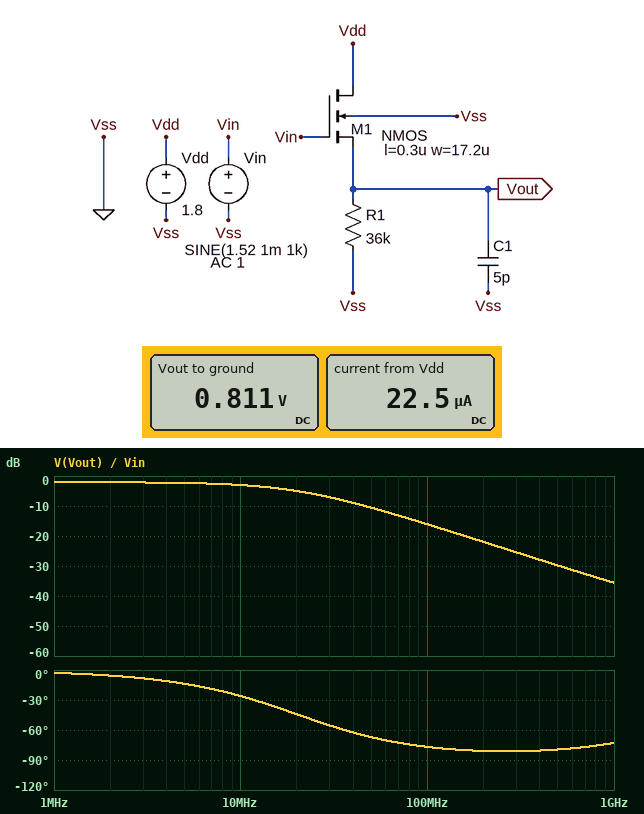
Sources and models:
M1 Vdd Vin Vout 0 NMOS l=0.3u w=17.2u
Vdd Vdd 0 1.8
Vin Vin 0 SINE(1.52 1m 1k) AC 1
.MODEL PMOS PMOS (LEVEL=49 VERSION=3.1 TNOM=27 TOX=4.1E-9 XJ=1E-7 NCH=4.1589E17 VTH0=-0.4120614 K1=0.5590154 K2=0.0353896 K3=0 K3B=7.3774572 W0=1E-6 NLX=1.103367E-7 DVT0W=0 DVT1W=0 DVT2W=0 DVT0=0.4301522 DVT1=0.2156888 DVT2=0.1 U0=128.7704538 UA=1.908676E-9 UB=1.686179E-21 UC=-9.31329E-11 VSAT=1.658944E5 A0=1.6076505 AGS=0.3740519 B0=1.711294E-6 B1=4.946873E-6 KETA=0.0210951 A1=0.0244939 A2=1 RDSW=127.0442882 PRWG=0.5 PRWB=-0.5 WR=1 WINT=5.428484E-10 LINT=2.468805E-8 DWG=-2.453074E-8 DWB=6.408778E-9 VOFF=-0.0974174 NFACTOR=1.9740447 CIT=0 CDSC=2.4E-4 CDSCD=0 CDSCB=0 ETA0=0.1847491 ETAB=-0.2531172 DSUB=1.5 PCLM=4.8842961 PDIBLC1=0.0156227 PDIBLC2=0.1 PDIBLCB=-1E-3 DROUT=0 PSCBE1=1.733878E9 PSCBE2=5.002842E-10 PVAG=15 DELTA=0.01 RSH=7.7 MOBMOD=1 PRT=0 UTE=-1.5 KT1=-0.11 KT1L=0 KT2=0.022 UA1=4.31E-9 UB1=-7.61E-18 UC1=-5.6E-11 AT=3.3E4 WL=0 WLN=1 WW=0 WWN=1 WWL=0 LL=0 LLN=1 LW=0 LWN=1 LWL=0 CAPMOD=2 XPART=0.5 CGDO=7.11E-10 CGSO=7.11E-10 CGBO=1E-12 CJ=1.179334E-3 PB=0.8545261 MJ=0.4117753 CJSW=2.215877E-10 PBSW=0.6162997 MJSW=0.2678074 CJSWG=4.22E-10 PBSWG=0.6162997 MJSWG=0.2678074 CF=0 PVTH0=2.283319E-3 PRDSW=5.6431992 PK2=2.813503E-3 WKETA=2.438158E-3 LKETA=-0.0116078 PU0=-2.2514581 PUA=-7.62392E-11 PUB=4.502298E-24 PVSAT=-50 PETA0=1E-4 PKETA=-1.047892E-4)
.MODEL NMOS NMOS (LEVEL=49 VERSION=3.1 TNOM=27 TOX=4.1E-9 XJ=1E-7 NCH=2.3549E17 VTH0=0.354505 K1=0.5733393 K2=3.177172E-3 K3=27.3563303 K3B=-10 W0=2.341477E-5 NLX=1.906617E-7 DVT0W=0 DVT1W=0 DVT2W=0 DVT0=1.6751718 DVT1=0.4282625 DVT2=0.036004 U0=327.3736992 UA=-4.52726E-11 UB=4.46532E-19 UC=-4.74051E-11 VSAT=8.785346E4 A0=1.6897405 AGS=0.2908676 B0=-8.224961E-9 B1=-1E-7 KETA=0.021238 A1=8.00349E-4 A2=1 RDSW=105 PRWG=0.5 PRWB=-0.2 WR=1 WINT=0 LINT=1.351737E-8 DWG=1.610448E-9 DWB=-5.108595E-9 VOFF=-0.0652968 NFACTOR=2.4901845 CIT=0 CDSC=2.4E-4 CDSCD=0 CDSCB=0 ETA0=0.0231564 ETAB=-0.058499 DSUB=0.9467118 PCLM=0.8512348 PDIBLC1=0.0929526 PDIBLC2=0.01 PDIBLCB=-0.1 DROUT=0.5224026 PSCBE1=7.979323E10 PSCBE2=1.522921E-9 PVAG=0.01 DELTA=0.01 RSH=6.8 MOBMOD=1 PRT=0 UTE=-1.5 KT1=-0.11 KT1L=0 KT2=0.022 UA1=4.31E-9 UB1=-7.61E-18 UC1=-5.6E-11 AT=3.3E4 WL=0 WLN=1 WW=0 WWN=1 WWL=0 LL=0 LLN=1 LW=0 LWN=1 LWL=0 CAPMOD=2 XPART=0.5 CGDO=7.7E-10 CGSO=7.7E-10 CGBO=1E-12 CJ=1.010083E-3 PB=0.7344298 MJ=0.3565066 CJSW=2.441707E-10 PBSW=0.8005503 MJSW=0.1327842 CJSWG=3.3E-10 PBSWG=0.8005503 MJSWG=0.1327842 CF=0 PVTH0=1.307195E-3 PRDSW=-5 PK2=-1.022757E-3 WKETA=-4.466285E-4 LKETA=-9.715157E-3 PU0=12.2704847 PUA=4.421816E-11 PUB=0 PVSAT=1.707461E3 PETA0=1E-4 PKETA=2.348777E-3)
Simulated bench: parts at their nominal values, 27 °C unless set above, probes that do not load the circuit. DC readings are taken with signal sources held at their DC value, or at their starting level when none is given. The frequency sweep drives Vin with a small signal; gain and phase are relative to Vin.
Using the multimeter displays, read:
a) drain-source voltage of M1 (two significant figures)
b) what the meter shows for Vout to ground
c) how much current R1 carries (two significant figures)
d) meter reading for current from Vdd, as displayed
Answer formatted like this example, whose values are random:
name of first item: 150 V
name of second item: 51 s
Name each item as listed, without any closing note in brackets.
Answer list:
drain-source voltage of M1: 990 mV
what the meter shows for Vout to ground: 0.811 V
how much current R1 carries: 23 µA
meter reading for current from Vdd, as displayed: 22.5 µA
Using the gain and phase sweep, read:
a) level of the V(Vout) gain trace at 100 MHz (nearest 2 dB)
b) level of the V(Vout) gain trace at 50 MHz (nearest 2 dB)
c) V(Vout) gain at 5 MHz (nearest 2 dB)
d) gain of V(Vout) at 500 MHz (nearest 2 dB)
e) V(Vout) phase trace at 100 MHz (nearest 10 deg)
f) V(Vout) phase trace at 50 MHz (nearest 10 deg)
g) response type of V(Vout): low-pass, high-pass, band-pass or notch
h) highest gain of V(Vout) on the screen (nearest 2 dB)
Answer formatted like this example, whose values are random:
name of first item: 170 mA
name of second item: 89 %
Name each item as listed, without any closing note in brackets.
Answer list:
level of the V(Vout) gain trace at 100 MHz: -16 dB
level of the V(Vout) gain trace at 50 MHz: -10 dB
V(Vout) gain at 5 MHz: -2 dB
gain of V(Vout) at 500 MHz: -30 dB
V(Vout) phase trace at 100 MHz: -80 deg
V(Vout) phase trace at 50 MHz: -70 deg
response type of V(Vout): low-pass, high-pass, band-pass or notch: low-pass
highest gain of V(Vout) on the screen: -2 dB
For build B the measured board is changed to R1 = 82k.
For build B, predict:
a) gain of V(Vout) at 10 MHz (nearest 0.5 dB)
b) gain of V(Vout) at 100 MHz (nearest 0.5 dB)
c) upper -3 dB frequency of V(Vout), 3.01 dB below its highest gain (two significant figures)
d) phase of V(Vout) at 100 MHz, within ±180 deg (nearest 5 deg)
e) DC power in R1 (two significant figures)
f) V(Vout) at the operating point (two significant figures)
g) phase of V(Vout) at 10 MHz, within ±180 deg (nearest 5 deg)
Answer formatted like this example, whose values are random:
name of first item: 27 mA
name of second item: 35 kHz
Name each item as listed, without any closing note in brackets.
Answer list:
gain of V(Vout) at 10 MHz: -5.0 dB
gain of V(Vout) at 100 MHz: -22.0 dB
upper -3 dB frequency of V(Vout), 3.01 dB below its highest gain: 9.9 MHz
phase of V(Vout) at 100 MHz, within ±180 deg: -80 deg
DC power in R1: 8.6 µW
V(Vout) at the operating point: 840 mV
phase of V(Vout) at 10 MHz, within ±180 deg: -45 deg
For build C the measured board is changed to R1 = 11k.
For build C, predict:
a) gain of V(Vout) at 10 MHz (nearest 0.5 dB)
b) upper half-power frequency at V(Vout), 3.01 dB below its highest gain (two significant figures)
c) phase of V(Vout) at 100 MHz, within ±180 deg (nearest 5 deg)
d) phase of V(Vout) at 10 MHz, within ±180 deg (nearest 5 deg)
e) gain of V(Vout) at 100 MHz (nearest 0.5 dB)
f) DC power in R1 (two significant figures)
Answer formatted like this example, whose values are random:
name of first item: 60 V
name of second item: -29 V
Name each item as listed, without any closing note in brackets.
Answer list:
gain of V(Vout) at 10 MHz: -2.5 dB
upper half-power frequency at V(Vout), 3.01 dB below its highest gain: 51 MHz
phase of V(Vout) at 100 MHz, within ±180 deg: -60 deg
phase of V(Vout) at 10 MHz, within ±180 deg: -10 deg
gain of V(Vout) at 100 MHz: -9.0 dB
DC power in R1: 53 µW
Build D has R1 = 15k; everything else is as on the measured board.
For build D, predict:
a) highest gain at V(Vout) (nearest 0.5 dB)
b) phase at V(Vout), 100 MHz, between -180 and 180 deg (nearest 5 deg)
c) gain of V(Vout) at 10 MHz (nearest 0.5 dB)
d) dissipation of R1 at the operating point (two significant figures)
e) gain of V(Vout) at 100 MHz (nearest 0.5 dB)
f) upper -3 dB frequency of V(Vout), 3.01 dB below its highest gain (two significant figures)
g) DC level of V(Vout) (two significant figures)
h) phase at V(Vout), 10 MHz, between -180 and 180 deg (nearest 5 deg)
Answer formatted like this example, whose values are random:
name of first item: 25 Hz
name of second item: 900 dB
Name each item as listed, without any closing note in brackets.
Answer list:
highest gain at V(Vout): -2.0 dB
phase at V(Vout), 100 MHz, between -180 and 180 deg: -65 deg
gain of V(Vout) at 10 MHz: -2.5 dB
dissipation of R1 at the operating point: 40 µW
gain of V(Vout) at 100 MHz: -10.5 dB
upper -3 dB frequency of V(Vout), 3.01 dB below its highest gain: 41 MHz
DC level of V(Vout): 780 mV
phase at V(Vout), 10 MHz, between -180 and 180 deg: -15 deg
